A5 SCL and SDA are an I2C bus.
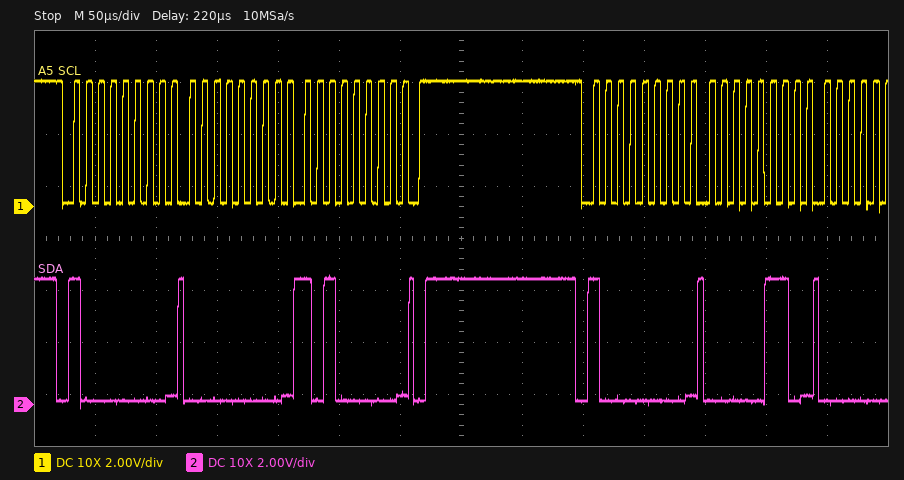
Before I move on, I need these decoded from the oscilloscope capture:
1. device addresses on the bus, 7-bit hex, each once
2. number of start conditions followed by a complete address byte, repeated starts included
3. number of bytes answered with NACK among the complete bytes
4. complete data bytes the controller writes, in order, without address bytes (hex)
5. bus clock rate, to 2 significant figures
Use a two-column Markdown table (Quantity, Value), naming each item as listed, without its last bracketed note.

| Quantity | Value |
|---|---|
| device addresses on the bus, 7-bit hex, each once | 0x40 |
| number of start conditions followed by a complete address byte, repeated starts included | 2 |
| number of bytes answered with NACK among the complete bytes | 0 |
| complete data bytes the controller writes, in order, without address bytes | 00 A0 06 |
| bus clock rate, to 2 significant figures | 100 kHz |
